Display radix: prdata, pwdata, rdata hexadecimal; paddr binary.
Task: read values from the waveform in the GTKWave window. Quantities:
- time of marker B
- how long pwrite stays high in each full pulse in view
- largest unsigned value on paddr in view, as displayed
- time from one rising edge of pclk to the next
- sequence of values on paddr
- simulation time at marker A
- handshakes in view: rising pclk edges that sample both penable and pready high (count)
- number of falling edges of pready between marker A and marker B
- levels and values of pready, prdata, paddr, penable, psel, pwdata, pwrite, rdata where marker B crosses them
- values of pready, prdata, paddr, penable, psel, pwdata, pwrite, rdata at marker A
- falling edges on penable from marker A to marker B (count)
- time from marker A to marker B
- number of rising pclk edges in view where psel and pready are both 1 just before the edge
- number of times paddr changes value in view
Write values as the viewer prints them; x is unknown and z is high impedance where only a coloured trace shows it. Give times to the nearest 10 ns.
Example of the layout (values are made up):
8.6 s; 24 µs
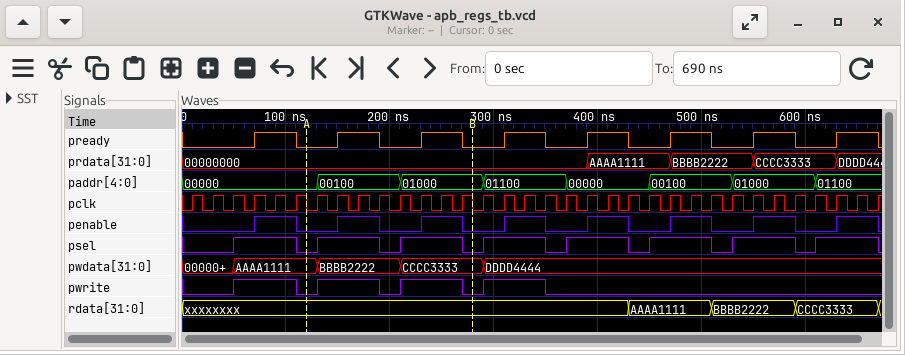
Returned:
280 ns; 60 ns, 60 ns, 60 ns, 60 ns; 01100; 20 ns; 00000, 00100, 01000, 01100, 00000, 00100, 01000, 01100; 120 ns; 16; 2; pready=0, prdata=00000000, paddr=01000, penable=0, psel=0, pwdata=CCCC3333, pwrite=0, rdata=xxxxxxxx; pready=0, prdata=00000000, paddr=00000, penable=0, psel=0, pwdata=AAAA1111, pwrite=0, rdata=xxxxxxxx; 2; 160 ns; 16; 7
